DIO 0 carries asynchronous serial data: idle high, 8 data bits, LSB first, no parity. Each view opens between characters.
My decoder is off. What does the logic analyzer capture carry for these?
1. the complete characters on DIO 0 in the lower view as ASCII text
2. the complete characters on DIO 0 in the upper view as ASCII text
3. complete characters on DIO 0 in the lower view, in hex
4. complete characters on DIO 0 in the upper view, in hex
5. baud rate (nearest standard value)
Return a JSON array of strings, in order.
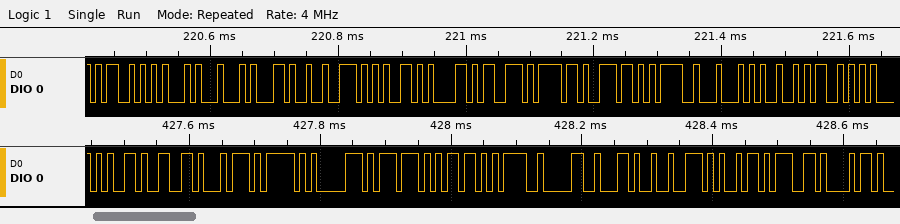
["\"eft_pwm=0,righ\"", "\"MED,reason=DIS\"", "65, 66, 74, 5F, 70, 77, 6D, 3D, 30, 2C, 72, 69, 67, 68", "4D, 45, 44, 2C, 72, 65, 61, 73, 6F, 6E, 3D, 44, 49, 53", "115200 baud"]
